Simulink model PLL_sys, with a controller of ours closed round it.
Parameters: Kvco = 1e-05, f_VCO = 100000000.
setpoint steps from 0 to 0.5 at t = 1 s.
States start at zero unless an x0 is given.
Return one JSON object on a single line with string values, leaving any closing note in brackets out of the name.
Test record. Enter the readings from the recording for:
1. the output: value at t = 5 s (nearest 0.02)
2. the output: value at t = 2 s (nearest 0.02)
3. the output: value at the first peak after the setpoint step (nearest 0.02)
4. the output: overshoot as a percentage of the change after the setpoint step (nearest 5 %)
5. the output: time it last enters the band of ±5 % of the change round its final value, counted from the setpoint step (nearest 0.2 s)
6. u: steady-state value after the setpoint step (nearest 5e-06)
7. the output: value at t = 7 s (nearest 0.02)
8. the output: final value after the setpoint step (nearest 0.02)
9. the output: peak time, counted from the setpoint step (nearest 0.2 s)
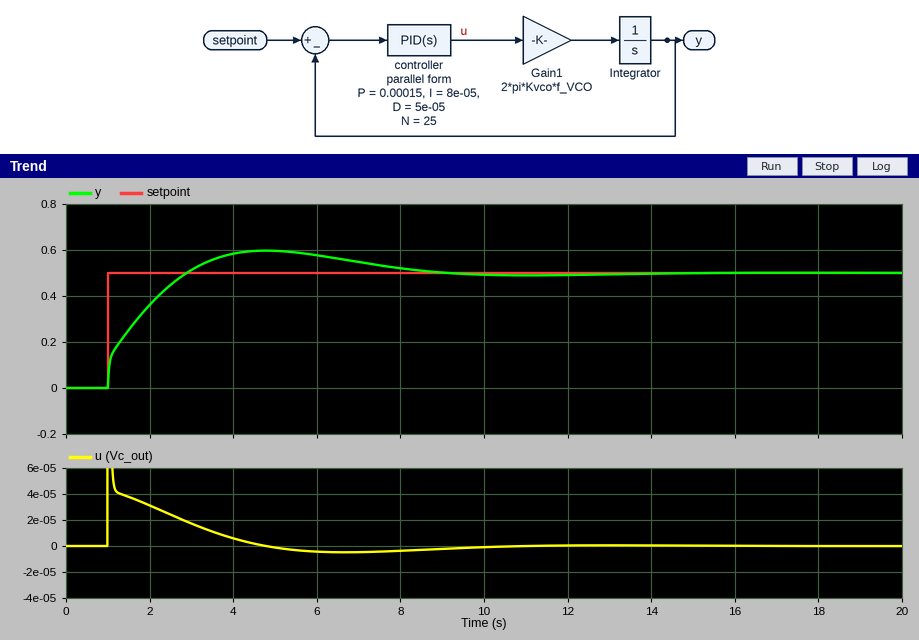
{"the output: value at t = 5 s": "0.60", "the output: value at t = 2 s": "0.36", "the output: value at the first peak after the setpoint step": "0.60", "the output: overshoot as a percentage of the change after the setpoint step": "20 %", "the output: time it last enters the band of ±5 % of the change round its final value, counted from the setpoint step": "6.8 s", "u: steady-state value after the setpoint step": "0.000000", "the output: value at t = 7 s": "0.54", "the output: final value after the setpoint step": "0.50", "the output: peak time, counted from the setpoint step": "3.8 s"}
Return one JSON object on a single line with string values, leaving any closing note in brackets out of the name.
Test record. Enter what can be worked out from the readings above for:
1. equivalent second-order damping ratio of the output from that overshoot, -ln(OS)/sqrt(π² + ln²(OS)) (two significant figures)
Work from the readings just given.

{"equivalent second-order damping ratio of the output from that overshoot, -ln(OS)/sqrt(π² + ln²(OS))": "0.46"}
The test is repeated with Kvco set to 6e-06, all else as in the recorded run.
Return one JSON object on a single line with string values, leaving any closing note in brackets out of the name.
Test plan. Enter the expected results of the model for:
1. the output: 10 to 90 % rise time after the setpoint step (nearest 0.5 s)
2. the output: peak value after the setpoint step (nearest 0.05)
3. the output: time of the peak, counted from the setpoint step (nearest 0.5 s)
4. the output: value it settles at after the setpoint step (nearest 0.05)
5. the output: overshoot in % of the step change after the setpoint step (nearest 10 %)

{"the output: 10 to 90 % rise time after the setpoint step": "2.0 s", "the output: peak value after the setpoint step": "0.65", "the output: time of the peak, counted from the setpoint step": "5.0 s", "the output: value it settles at after the setpoint step": "0.50", "the output: overshoot in % of the step change after the setpoint step": "30 %"}
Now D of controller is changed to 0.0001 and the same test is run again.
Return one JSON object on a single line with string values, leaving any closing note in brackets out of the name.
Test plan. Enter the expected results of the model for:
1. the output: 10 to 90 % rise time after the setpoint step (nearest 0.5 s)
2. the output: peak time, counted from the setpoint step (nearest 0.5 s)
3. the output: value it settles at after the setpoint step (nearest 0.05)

{"the output: 10 to 90 % rise time after the setpoint step": "1.5 s", "the output: peak time, counted from the setpoint step": "4.5 s", "the output: value it settles at after the setpoint step": "0.50"}
